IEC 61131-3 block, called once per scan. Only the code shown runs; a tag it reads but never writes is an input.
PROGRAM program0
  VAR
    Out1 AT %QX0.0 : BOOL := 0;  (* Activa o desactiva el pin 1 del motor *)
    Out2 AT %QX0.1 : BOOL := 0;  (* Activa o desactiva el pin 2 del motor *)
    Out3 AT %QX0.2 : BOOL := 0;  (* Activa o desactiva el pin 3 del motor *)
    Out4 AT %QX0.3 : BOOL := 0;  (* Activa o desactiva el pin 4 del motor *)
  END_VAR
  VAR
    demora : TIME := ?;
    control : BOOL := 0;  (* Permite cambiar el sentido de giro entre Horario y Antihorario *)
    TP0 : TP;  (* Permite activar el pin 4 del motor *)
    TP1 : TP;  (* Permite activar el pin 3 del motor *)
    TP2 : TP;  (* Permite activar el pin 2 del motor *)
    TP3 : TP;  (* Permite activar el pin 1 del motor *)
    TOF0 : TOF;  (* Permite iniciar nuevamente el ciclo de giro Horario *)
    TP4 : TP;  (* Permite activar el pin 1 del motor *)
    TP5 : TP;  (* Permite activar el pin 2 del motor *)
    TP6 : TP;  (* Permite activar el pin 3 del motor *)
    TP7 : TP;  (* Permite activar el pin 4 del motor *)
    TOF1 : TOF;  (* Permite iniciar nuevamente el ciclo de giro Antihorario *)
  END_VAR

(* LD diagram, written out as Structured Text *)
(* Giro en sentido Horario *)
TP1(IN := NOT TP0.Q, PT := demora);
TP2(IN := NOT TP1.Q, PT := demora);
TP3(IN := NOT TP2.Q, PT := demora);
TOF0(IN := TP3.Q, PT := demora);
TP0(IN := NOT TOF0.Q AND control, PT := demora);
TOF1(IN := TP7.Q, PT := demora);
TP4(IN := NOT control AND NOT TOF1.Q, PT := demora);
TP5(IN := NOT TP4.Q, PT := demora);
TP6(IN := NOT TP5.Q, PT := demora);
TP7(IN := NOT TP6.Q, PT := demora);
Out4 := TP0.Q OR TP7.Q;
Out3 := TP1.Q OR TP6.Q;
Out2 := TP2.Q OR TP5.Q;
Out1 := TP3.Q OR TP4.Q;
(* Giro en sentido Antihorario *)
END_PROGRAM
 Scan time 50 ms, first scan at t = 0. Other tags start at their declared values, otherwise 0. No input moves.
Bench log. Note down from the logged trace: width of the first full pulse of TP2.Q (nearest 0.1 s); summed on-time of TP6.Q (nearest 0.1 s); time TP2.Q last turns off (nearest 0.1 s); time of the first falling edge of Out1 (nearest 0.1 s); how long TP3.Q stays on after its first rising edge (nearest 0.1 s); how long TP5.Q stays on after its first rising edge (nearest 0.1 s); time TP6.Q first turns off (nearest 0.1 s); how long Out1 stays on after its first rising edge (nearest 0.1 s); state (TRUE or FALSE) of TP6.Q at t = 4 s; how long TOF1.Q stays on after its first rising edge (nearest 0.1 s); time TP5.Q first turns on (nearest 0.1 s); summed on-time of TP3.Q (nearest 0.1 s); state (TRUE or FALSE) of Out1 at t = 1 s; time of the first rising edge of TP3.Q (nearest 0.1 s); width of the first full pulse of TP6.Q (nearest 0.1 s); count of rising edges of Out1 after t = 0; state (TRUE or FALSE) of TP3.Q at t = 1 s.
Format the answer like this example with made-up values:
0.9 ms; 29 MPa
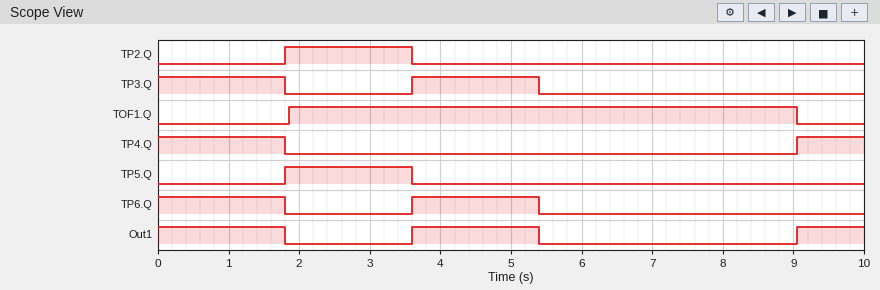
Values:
1.8 s; 3.6 s; 3.6 s; 1.8 s; 1.8 s; 1.8 s; 1.8 s; 1.8 s; TRUE; 7.2 s; 1.8 s; 3.6 s; TRUE; 3.6 s; 1.8 s; 2; TRUE
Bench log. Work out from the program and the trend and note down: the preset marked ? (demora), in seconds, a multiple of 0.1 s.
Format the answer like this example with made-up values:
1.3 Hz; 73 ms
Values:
1.8 s
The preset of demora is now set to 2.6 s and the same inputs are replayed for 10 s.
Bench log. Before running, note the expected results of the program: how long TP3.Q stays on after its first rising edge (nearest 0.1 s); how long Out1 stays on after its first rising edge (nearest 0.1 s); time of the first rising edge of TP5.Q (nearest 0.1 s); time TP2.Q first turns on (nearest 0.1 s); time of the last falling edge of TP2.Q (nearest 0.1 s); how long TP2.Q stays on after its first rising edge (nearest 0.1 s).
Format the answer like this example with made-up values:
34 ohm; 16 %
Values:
2.6 s; 2.6 s; 2.6 s; 2.6 s; 5.2 s; 2.6 s
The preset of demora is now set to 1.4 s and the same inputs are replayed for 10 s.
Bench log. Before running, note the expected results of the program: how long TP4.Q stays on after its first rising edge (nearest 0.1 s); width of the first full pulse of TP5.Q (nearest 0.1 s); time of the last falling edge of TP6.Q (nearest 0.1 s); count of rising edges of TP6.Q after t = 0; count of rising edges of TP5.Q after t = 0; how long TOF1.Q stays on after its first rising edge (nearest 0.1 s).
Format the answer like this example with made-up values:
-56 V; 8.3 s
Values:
1.4 s; 1.4 s; 4.2 s; 2; 2; 5.6 s
